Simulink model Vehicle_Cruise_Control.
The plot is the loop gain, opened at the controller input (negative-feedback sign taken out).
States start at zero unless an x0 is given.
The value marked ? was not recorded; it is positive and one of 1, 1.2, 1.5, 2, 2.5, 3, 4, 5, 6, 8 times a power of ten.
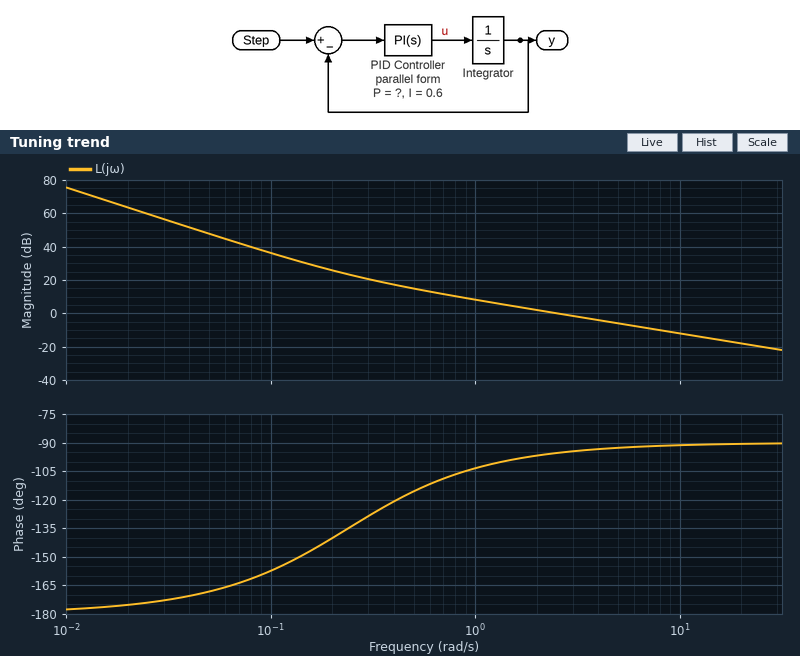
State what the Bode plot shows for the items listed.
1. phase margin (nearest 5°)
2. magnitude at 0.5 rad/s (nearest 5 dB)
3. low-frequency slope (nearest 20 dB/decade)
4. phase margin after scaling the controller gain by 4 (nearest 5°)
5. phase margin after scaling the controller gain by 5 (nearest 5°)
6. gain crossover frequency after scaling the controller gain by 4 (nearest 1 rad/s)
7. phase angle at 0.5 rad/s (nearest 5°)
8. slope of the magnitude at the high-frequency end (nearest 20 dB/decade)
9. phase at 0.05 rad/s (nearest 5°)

85°
15 dB
-40 dB/decade
90°
90°
10 rad/s
-115°
-20 dB/decade
-170°
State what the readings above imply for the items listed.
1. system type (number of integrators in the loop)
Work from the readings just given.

2
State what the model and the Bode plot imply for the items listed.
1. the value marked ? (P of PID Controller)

2.5
